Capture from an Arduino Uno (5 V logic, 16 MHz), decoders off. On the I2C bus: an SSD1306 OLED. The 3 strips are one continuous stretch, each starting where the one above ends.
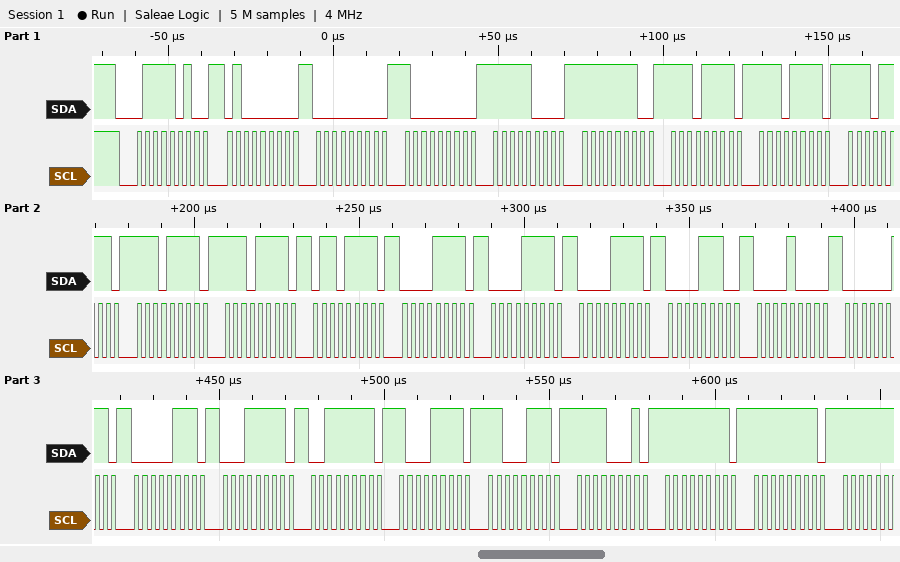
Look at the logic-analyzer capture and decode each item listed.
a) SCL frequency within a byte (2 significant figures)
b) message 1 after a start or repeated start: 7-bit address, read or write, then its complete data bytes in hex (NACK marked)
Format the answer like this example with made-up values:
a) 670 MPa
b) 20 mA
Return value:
a) 400 kHz
b) 0x3D write: 40 00 80 F8 FE EF EF EF EF EF 6F 0F 0F 0F 0E 08 03 07 1F 3F 8F C7 F1 FF FF
